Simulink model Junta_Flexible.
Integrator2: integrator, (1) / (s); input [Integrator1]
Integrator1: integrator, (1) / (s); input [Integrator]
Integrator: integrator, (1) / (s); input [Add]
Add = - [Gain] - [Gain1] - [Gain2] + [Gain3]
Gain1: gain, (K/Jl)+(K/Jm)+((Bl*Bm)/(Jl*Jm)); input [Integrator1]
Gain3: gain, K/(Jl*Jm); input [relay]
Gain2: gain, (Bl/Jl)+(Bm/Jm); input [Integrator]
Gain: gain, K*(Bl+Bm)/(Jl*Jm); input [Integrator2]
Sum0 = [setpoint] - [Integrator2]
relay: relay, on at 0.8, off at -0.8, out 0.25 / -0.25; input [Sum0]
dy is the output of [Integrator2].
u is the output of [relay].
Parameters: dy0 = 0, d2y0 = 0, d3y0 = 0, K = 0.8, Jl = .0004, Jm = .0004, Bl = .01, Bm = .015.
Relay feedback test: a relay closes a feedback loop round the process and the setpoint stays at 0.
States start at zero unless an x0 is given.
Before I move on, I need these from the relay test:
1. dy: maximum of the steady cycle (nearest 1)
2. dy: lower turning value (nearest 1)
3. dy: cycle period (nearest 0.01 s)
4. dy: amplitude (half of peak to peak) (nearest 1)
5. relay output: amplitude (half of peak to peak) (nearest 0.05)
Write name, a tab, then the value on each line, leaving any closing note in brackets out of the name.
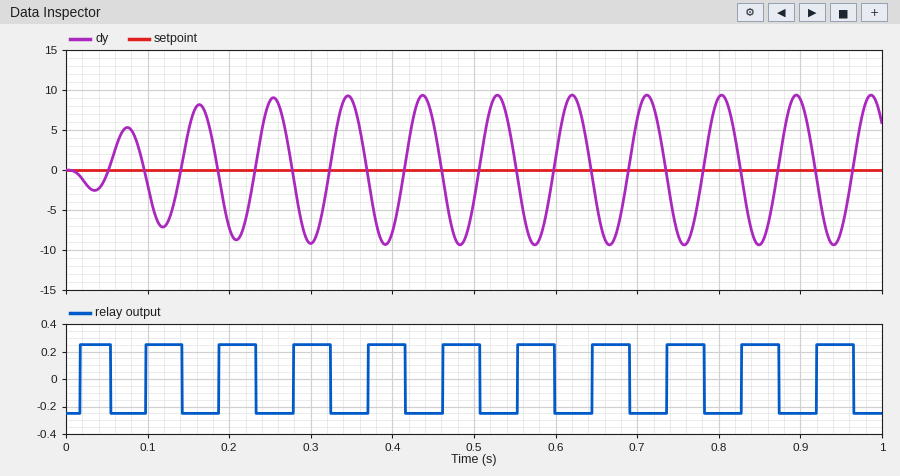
dy: maximum of the steady cycle	9
dy: lower turning value	-9
dy: cycle period	0.09 s
dy: amplitude (half of peak to peak)	9
relay output: amplitude (half of peak to peak)	0.25
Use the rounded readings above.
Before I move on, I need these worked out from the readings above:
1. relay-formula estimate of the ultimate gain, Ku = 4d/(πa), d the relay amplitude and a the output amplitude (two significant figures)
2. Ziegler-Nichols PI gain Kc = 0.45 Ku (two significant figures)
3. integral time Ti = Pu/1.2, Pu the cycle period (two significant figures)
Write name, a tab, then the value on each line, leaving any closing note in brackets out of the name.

relay-formula estimate of the ultimate gain, Ku = 4d/(πa), d the relay amplitude and a the output amplitude	0.035
Ziegler-Nichols PI gain Kc = 0.45 Ku	0.016
integral time Ti = Pu/1.2, Pu the cycle period	0.075 s
